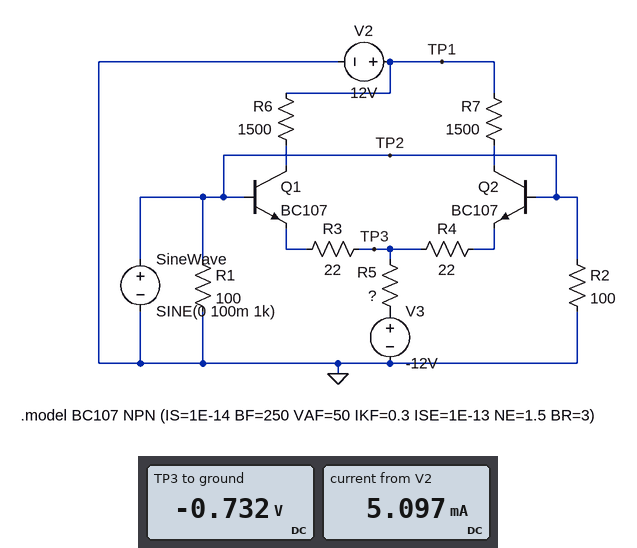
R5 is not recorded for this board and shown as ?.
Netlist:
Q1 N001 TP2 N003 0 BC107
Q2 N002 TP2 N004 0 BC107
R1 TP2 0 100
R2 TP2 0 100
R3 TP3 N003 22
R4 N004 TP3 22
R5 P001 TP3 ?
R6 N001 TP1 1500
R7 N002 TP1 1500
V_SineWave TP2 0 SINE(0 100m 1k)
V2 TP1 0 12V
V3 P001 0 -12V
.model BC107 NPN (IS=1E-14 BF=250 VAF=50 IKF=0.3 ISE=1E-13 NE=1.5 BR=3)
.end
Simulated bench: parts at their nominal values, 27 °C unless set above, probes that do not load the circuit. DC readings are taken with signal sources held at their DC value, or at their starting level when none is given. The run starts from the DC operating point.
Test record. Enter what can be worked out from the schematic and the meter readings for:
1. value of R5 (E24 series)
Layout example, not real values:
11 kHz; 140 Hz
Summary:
2.2 kΩ
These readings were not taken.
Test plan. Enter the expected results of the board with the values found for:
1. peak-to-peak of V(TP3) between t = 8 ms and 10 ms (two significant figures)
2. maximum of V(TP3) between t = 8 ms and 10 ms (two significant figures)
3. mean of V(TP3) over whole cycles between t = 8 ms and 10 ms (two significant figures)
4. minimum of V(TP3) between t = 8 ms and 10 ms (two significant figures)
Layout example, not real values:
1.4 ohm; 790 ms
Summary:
200 mV; -630 mV; -730 mV; -830 mV
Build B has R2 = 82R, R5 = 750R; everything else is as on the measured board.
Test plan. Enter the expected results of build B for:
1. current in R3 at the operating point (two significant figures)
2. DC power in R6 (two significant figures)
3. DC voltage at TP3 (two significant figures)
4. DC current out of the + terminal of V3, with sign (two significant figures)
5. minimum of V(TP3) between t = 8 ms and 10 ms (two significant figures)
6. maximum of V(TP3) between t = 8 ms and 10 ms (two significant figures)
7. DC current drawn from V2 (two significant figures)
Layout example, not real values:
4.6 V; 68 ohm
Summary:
7.4 mA; 82 mW; -870 mV; -15 mA; -970 mV; -770 mV; 15 mA
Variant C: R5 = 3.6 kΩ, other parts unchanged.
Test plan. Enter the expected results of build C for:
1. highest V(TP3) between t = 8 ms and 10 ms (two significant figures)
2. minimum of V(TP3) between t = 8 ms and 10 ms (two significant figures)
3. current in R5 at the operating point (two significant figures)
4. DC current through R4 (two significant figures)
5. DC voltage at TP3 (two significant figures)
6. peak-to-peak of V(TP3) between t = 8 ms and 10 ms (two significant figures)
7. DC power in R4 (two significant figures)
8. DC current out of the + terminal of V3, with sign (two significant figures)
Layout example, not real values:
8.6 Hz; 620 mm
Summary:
-600 mV; -800 mV; 3.1 mA; 1.6 mA; -700 mV; 200 mV; 54 µW; -3.1 mA
